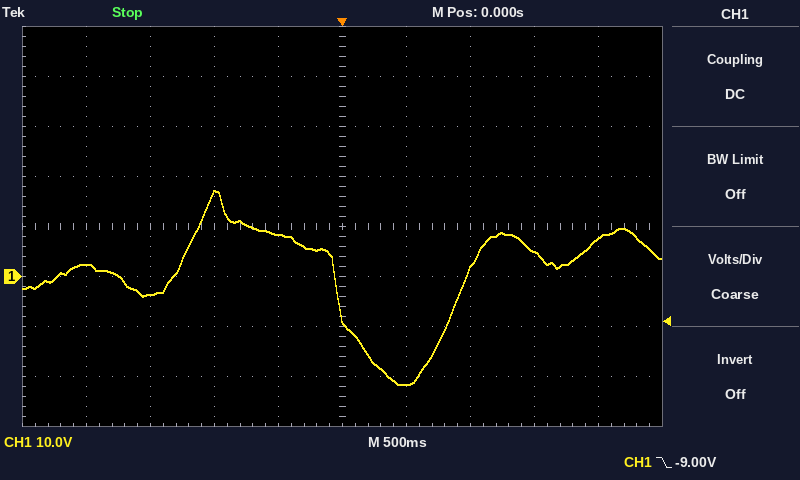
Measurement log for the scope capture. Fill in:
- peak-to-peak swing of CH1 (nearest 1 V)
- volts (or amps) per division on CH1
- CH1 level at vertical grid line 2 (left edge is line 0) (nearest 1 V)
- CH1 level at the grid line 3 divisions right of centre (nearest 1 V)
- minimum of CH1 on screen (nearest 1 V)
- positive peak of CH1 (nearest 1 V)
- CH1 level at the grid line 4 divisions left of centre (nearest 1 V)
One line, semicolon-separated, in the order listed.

39 V; 10 V; -4 V; 5 V; -22 V; 17 V; 2 V
